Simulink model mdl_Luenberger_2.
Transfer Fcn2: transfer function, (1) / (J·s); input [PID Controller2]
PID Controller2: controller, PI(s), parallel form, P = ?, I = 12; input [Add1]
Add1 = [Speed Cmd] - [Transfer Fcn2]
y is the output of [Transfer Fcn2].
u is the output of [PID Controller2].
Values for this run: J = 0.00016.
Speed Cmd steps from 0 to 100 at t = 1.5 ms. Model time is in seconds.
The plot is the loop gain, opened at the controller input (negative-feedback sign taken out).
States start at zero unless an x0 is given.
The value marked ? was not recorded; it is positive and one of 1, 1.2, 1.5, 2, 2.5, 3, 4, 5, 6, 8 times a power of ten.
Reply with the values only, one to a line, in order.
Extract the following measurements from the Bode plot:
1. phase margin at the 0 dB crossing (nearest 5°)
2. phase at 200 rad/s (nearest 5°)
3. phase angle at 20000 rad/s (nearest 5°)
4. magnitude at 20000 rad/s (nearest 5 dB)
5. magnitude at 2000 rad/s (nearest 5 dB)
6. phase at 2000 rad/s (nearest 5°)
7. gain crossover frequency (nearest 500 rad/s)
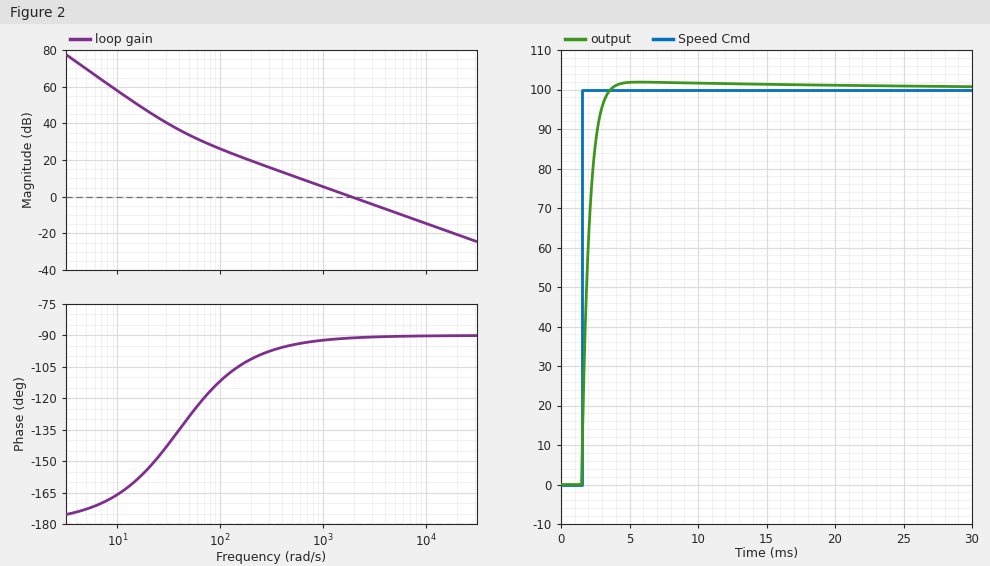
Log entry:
90°
-100°
-90°
-20 dB
0 dB
-90°
2000 rad/s
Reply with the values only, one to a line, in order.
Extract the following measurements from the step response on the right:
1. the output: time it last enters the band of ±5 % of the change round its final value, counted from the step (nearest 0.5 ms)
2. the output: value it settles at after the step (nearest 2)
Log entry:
1.5 ms
100
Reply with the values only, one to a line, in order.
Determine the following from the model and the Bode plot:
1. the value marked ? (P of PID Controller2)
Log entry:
0.3
